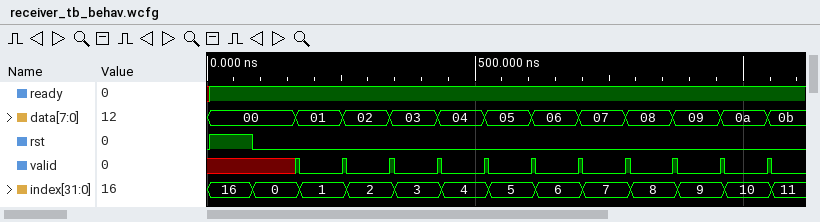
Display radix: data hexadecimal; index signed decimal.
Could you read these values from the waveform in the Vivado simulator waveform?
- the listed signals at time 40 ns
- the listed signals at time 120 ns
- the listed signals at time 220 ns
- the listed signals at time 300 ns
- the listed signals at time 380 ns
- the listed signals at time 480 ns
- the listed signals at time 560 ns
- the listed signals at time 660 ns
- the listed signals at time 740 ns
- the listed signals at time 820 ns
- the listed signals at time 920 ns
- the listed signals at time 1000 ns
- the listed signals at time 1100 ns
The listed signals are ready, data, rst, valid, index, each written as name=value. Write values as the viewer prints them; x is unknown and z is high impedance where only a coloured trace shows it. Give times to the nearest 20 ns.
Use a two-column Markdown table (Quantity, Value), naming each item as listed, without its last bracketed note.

| Quantity | Value |
|---|---|
| the listed signals at time 40 ns | ready=1, data=00, rst=1, valid=x, index=16 |
| the listed signals at time 120 ns | ready=1, data=00, rst=0, valid=x, index=0 |
| the listed signals at time 220 ns | ready=1, data=01, rst=0, valid=0, index=1 |
| the listed signals at time 300 ns | ready=1, data=02, rst=0, valid=0, index=2 |
| the listed signals at time 380 ns | ready=1, data=03, rst=0, valid=0, index=3 |
| the listed signals at time 480 ns | ready=1, data=04, rst=0, valid=0, index=4 |
| the listed signals at time 560 ns | ready=1, data=05, rst=0, valid=0, index=5 |
| the listed signals at time 660 ns | ready=1, data=06, rst=0, valid=0, index=6 |
| the listed signals at time 740 ns | ready=1, data=07, rst=0, valid=0, index=7 |
| the listed signals at time 820 ns | ready=1, data=08, rst=0, valid=0, index=8 |
| the listed signals at time 920 ns | ready=1, data=09, rst=0, valid=0, index=9 |
| the listed signals at time 1000 ns | ready=1, data=0a, rst=0, valid=0, index=10 |
| the listed signals at time 1100 ns | ready=1, data=0b, rst=0, valid=0, index=11 |
